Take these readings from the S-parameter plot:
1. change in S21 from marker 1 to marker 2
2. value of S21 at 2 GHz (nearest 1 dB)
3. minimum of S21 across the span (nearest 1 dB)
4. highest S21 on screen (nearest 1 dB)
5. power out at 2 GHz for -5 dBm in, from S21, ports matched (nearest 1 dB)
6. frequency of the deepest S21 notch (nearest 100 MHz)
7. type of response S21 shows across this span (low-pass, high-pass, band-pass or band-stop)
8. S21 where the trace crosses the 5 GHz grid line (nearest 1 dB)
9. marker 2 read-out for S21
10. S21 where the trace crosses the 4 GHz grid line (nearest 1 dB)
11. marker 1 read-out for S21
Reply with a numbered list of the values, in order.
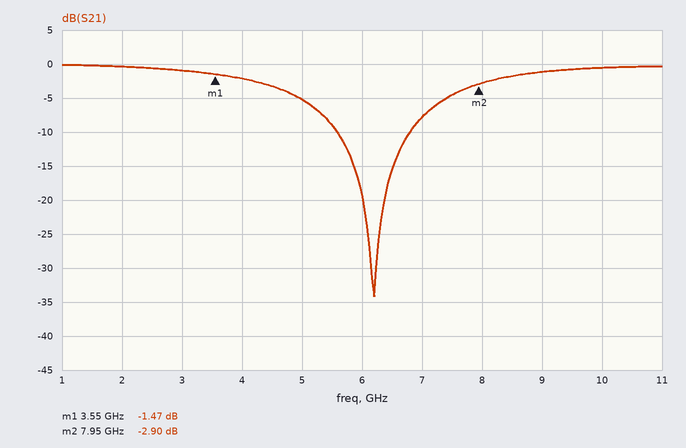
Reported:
1. -1.43 dB
2. 0 dB
3. -34 dB
4. 0 dB
5. -5 dBm
6. 6.2 GHz
7. band-stop
8. -5 dB
9. -2.90 dB
10. -2 dB
11. -1.47 dB
